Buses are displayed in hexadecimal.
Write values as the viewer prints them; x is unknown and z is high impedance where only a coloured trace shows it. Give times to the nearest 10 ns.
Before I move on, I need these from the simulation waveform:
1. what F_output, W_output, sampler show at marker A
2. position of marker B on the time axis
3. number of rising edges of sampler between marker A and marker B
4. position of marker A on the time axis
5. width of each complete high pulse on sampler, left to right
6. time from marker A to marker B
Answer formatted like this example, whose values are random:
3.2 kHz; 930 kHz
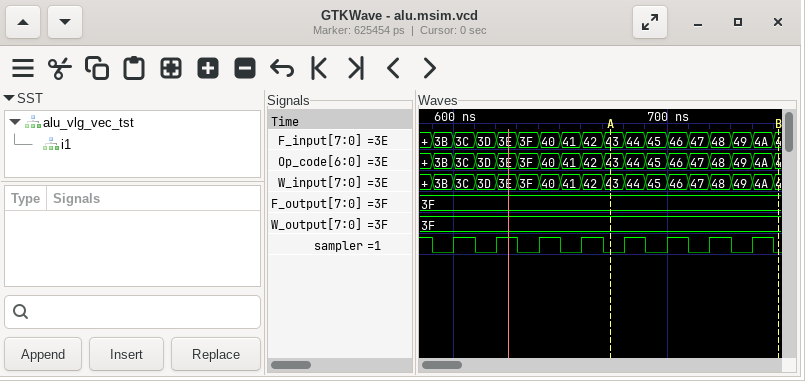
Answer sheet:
F_output=3F, W_output=3F, sampler=0; 750 ns; 4; 670 ns; 10 ns, 10 ns, 10 ns, 10 ns, 10 ns, 10 ns, 10 ns, 10 ns; 80 ns
